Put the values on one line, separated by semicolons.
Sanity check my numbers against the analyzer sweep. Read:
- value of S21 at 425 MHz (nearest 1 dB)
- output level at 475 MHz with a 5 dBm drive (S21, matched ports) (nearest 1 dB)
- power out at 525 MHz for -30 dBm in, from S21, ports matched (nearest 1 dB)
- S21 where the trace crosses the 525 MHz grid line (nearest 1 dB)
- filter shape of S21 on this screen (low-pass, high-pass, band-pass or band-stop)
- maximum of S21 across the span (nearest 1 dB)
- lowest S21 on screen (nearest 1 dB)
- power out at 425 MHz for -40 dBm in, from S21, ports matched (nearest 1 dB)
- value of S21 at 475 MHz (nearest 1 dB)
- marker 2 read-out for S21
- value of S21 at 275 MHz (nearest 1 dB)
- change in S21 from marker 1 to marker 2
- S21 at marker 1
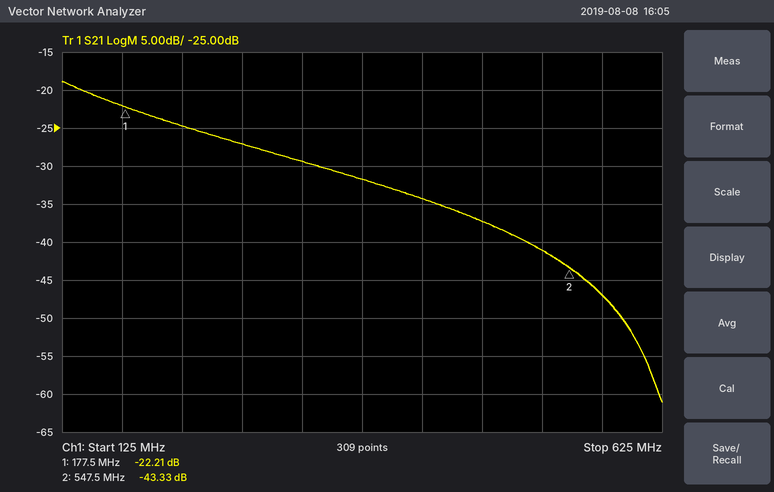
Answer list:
-34 dB; -32 dBm; -71 dBm; -41 dB; low-pass; -19 dB; -61 dB; -74 dBm; -37 dB; -43.33 dB; -27 dB; -21.12 dB; -22.21 dB
